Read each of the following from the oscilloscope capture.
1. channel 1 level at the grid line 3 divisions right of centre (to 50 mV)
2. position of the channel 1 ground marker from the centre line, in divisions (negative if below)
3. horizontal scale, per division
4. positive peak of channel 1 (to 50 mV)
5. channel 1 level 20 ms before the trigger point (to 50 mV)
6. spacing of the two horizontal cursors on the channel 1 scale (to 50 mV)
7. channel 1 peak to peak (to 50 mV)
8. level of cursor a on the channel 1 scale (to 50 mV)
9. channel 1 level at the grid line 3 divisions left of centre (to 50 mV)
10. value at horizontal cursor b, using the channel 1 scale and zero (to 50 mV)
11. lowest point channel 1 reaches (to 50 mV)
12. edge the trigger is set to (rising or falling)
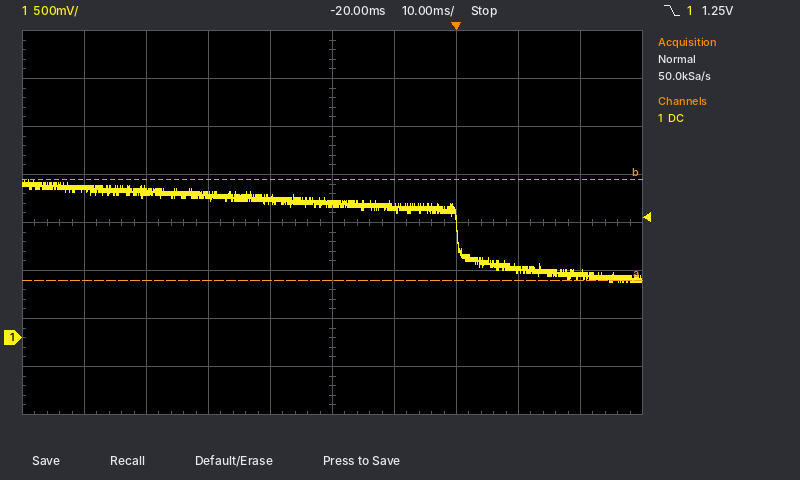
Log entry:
700 mV
-2.4 div
10 ms
1.65 V
1.40 V
1.05 V
1.05 V
600 mV
1.55 V
1.65 V
600 mV
falling
